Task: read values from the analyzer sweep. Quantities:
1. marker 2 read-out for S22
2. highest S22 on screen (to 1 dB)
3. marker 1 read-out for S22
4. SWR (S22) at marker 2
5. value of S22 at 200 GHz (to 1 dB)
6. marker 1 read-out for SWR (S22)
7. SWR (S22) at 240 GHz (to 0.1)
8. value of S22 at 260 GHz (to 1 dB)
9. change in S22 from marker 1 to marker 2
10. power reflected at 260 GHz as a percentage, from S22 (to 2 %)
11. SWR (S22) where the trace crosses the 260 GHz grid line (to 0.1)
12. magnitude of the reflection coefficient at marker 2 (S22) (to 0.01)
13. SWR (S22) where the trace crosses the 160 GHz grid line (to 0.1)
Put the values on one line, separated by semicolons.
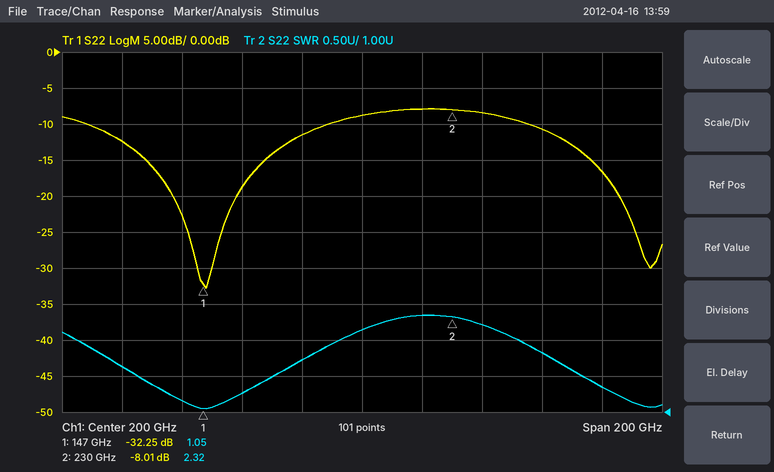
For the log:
-8.01 dB; -8 dB; -32.25 dB; 2.32; -9 dB; 1.05; 2.2; -11 dB; 24.24 dB; 8 %; 1.8; 0.40; 1.3
